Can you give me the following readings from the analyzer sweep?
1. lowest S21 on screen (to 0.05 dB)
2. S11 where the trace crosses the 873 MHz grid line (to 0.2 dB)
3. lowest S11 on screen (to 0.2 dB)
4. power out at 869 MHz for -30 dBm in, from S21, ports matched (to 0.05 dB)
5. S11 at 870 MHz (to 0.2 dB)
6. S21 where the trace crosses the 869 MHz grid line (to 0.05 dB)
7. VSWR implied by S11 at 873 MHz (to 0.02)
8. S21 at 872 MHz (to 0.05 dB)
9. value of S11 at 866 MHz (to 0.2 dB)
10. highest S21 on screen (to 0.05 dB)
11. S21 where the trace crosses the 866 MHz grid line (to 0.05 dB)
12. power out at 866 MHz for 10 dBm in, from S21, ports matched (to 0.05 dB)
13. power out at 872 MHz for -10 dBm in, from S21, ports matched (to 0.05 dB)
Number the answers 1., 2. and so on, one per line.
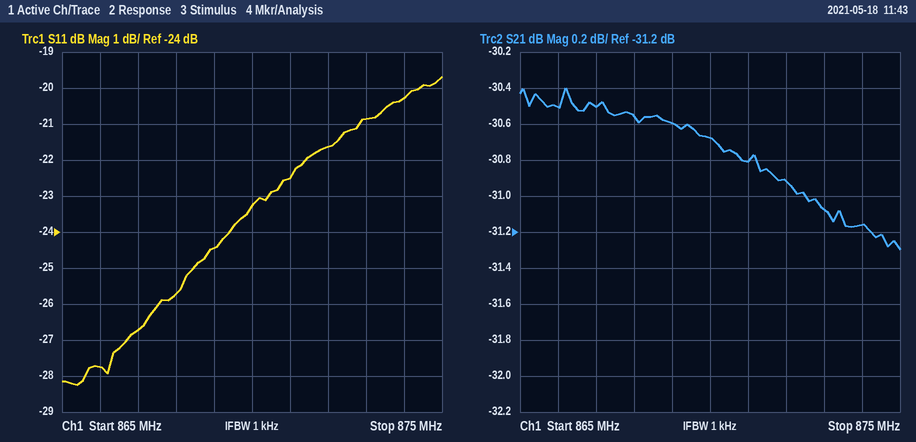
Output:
1. -31.30 dB
2. -20.8 dB
3. -28.2 dB
4. -60.60 dBm
5. -23.2 dB
6. -30.60 dB
7. 1.20
8. -30.90 dB
9. -27.8 dB
10. -30.40 dB
11. -30.50 dB
12. -20.50 dBm
13. -40.90 dBm
